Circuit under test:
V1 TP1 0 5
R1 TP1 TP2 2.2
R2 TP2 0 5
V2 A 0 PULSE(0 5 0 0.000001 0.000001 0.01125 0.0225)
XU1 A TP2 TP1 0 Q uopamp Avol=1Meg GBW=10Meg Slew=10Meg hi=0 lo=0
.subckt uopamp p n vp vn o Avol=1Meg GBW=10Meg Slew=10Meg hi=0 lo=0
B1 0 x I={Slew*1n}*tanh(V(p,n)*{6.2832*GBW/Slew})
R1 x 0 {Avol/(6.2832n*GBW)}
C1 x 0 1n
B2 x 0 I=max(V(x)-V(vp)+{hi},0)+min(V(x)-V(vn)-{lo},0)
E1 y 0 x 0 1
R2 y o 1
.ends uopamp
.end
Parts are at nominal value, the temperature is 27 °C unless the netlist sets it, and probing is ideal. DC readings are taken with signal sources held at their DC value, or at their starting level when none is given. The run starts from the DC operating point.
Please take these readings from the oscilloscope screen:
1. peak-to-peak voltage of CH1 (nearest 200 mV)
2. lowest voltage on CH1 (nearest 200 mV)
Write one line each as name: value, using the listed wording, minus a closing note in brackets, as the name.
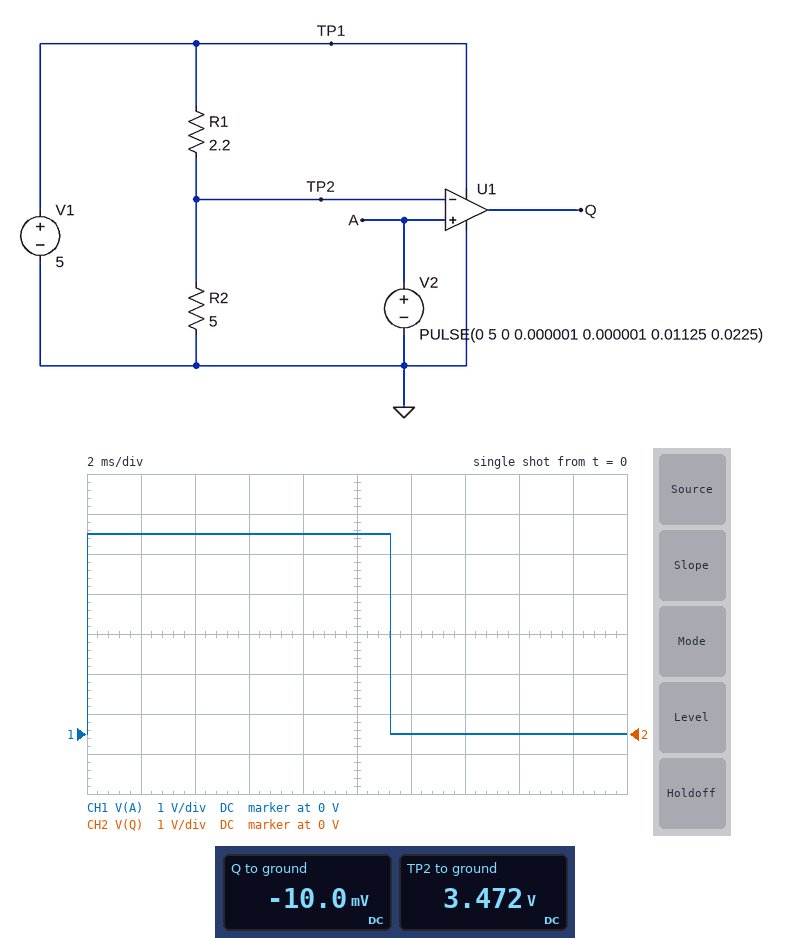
peak-to-peak voltage of CH1: 5.0 V
lowest voltage on CH1: 0 V
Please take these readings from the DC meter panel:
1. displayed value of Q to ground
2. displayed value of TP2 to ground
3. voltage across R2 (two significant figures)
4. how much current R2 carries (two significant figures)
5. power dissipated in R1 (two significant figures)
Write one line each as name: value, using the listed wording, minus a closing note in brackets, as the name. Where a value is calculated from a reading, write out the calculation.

displayed value of Q to ground: -10.0 mV
displayed value of TP2 to ground: 3.472 V
voltage across R2: 3.472 V = 3.5 V
how much current R2 carries: (3.472 V) / 5 Ω = 690 mA
power dissipated in R1: (5 V - 3.472 V)^2 / 2.2 Ω = 1.1 W
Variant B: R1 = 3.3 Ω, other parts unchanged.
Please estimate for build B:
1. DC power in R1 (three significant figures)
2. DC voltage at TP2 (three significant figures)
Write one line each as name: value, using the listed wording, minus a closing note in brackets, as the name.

DC power in R1: 1.20 W
DC voltage at TP2: 3.01 V
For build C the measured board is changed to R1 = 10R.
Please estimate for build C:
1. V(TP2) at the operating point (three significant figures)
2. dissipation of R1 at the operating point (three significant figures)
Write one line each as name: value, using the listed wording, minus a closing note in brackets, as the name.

V(TP2) at the operating point: 1.67 V
dissipation of R1 at the operating point: 1.11 W
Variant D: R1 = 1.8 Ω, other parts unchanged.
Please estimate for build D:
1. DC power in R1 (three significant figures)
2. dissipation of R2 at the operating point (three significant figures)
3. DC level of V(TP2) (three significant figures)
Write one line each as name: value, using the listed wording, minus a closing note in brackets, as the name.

DC power in R1: 973 mW
dissipation of R2 at the operating point: 2.70 W
DC level of V(TP2): 3.68 V
